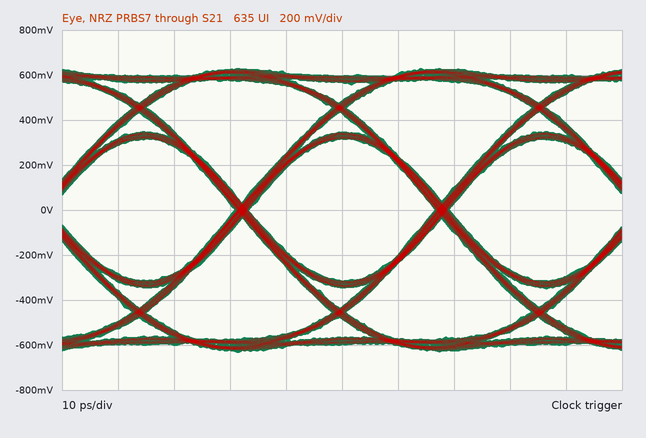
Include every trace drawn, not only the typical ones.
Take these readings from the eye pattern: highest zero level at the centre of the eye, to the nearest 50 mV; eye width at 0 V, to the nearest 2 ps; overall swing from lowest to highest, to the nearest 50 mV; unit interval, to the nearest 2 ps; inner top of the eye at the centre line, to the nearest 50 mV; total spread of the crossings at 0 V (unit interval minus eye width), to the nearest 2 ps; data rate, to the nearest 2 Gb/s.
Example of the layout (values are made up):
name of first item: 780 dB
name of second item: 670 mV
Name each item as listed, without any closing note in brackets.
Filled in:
highest zero level at the centre of the eye, to the nearest 50 mV: -300 mV
eye width at 0 V, to the nearest 2 ps: 34 ps
overall swing from lowest to highest, to the nearest 50 mV: 1.25 V
unit interval, to the nearest 2 ps: 36 ps
inner top of the eye at the centre line, to the nearest 50 mV: 300 mV
total spread of the crossings at 0 V (unit interval minus eye width), to the nearest 2 ps: 2 ps
data rate, to the nearest 2 Gb/s: 28 Gb/s
